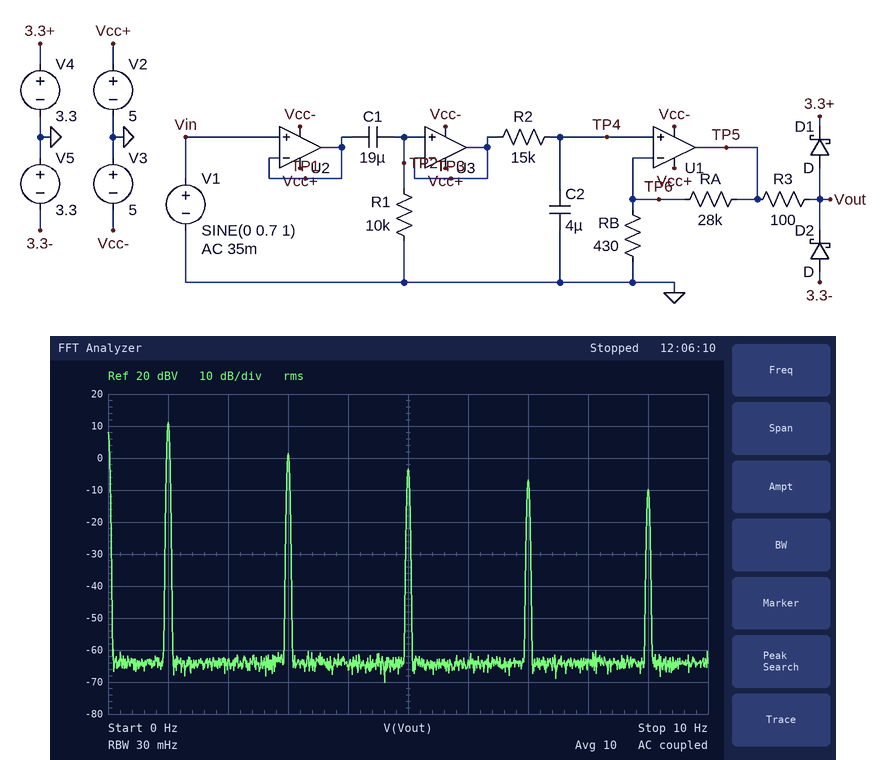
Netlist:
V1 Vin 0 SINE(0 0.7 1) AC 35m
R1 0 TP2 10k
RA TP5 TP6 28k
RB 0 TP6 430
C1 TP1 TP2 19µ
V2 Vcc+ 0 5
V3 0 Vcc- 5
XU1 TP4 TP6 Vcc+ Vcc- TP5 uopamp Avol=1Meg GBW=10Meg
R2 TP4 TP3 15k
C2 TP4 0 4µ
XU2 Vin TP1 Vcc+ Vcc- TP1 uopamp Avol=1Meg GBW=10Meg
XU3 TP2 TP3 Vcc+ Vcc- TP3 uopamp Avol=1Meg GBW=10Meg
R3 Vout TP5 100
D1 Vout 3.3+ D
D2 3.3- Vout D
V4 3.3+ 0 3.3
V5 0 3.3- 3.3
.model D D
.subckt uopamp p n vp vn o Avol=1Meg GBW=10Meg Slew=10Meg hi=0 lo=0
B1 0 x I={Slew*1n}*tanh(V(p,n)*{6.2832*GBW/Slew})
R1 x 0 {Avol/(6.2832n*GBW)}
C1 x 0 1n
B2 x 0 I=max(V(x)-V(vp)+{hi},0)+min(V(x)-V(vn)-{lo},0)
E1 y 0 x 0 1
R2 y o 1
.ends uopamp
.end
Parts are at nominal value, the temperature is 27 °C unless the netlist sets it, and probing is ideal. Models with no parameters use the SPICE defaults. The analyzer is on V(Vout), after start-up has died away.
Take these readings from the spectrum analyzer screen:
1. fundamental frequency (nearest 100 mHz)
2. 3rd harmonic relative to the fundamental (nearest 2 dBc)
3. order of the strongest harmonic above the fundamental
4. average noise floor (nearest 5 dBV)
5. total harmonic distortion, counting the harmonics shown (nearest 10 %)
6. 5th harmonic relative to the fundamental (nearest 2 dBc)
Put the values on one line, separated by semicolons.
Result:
1.0 Hz; -10 dBc; 3; -65 dBV; 40 %; -14 dBc
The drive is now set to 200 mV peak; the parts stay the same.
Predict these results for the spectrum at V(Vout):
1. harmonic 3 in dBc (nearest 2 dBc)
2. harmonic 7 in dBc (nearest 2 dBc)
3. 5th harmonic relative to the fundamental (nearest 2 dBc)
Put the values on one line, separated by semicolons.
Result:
-12 dBc; -44 dBc; -22 dBc
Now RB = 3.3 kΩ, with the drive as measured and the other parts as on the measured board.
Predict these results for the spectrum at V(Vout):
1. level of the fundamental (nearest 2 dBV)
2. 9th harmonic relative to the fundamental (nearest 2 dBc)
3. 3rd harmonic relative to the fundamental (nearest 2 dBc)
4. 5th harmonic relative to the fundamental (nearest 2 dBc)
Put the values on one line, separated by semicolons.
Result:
10 dBV; -44 dBc; -24 dBc; -30 dBc
